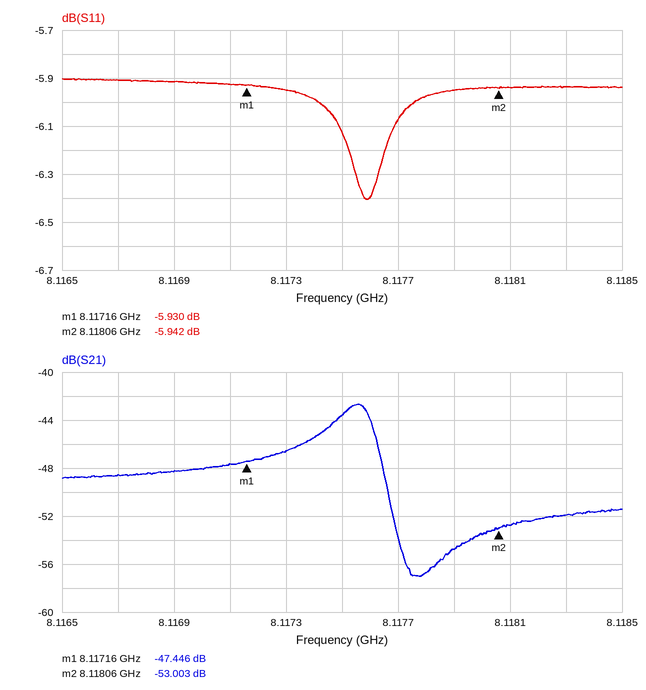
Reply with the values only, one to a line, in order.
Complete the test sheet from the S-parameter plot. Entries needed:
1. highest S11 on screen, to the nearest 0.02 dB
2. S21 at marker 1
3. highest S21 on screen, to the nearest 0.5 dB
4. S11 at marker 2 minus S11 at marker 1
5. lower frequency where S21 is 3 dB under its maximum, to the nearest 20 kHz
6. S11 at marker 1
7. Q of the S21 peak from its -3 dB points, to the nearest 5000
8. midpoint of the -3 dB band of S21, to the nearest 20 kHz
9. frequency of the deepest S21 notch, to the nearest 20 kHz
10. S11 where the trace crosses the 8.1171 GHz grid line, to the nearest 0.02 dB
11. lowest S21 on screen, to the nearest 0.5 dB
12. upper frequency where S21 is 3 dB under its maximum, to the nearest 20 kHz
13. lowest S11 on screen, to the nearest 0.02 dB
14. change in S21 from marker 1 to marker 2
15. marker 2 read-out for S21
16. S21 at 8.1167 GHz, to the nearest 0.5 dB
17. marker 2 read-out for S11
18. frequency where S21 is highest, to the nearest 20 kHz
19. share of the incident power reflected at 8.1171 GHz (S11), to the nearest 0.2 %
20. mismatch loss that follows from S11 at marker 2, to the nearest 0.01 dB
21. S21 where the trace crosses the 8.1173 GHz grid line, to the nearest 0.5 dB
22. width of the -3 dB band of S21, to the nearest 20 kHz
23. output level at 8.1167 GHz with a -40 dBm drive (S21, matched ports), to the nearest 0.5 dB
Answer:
-5.90 dB
-47.446 dB
-42.5 dB
-0.012 dB
8.11738 GHz
-5.930 dB
35000
8.11750 GHz
8.11778 GHz
-5.92 dB
-57.0 dB
8.11762 GHz
-6.40 dB
-5.557 dB
-53.003 dB
-48.5 dB
-5.942 dB
8.11756 GHz
25.6 %
1.28 dB
-46.5 dB
240 kHz
-88.5 dBm
